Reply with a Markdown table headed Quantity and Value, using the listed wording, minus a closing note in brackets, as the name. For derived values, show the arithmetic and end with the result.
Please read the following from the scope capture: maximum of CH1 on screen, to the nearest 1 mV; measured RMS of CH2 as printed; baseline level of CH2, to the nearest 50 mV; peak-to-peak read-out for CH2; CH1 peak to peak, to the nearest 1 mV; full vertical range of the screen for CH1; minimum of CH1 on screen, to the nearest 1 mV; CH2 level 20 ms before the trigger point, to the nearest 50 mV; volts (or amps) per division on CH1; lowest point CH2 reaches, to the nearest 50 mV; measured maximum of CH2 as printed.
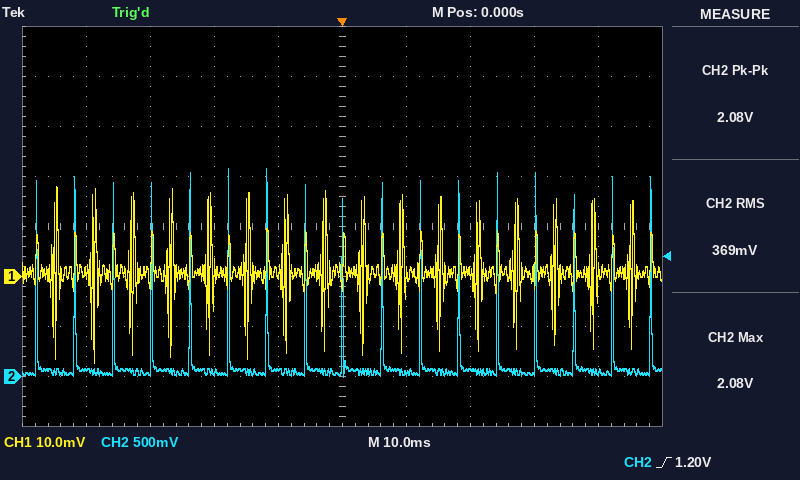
| Quantity | Value |
|---|---|
| maximum of CH1 on screen, to the nearest 1 mV | 18 mV |
| measured RMS of CH2 as printed | 369 mV |
| baseline level of CH2, to the nearest 50 mV | 50 mV |
| peak-to-peak read-out for CH2 | 2.08 V |
| CH1 peak to peak, to the nearest 1 mV | 18 mV − (-17 mV) = 35 mV |
| full vertical range of the screen for CH1 | 80 mV |
| minimum of CH1 on screen, to the nearest 1 mV | -17 mV |
| CH2 level 20 ms before the trigger point, to the nearest 50 mV | 50 mV |
| volts (or amps) per division on CH1 | 10 mV |
| lowest point CH2 reaches, to the nearest 50 mV | 0 mV |
| measured maximum of CH2 as printed | 2.08 V |
